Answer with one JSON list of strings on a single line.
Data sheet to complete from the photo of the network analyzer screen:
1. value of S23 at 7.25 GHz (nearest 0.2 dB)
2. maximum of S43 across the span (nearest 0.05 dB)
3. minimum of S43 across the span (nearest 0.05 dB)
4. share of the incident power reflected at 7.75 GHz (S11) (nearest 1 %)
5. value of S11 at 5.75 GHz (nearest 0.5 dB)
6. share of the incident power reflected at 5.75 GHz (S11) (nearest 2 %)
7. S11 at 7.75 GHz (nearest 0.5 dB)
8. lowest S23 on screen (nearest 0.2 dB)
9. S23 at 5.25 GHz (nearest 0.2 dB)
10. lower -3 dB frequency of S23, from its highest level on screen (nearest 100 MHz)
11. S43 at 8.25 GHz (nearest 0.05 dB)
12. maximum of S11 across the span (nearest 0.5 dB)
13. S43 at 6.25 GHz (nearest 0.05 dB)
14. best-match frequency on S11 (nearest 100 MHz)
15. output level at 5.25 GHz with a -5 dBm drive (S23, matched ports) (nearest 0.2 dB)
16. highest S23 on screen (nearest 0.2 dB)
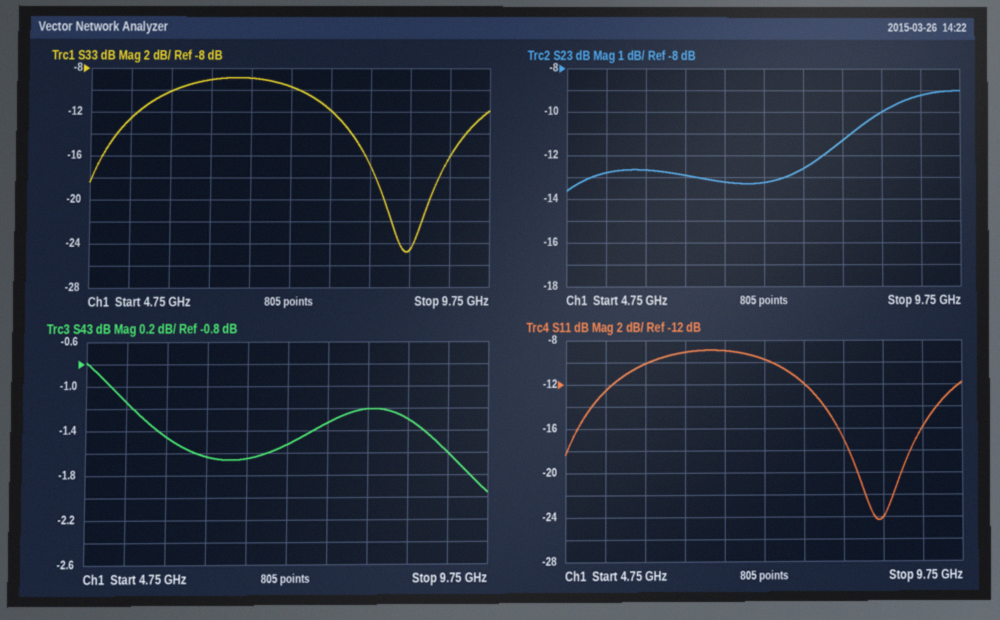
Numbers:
["-13.2 dB", "-0.80 dB", "-1.95 dB", "6 %", "-10.0 dB", "10 %", "-12.0 dB", "-13.6 dB", "-12.8 dB", "8.0 GHz", "-1.20 dB", "-9.0 dB", "-1.65 dB", "8.7 GHz", "-17.8 dBm", "-9.0 dB"]
